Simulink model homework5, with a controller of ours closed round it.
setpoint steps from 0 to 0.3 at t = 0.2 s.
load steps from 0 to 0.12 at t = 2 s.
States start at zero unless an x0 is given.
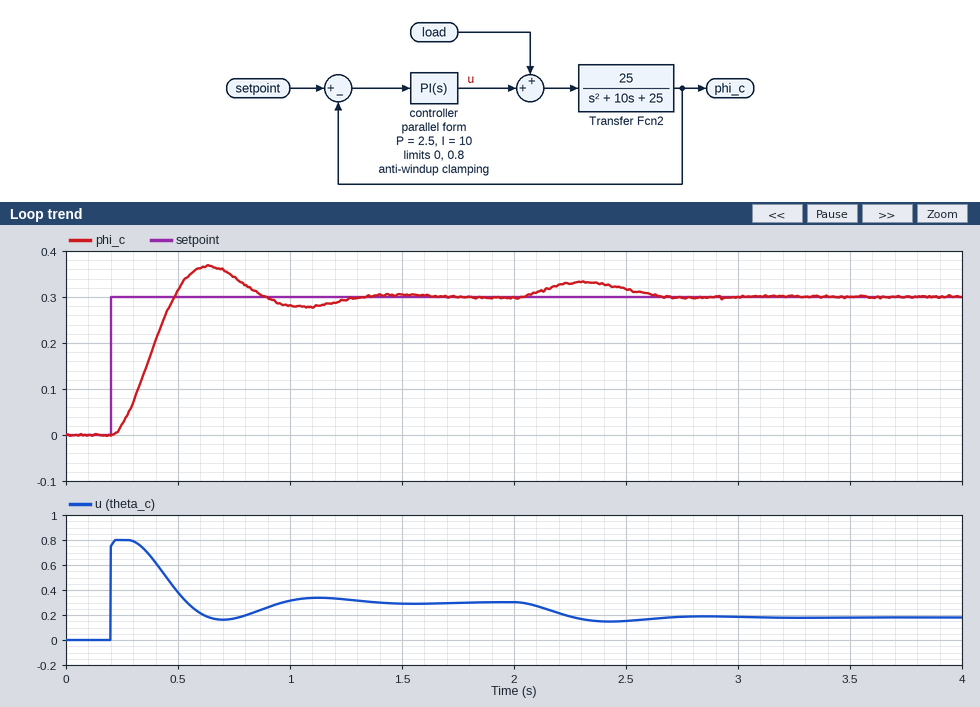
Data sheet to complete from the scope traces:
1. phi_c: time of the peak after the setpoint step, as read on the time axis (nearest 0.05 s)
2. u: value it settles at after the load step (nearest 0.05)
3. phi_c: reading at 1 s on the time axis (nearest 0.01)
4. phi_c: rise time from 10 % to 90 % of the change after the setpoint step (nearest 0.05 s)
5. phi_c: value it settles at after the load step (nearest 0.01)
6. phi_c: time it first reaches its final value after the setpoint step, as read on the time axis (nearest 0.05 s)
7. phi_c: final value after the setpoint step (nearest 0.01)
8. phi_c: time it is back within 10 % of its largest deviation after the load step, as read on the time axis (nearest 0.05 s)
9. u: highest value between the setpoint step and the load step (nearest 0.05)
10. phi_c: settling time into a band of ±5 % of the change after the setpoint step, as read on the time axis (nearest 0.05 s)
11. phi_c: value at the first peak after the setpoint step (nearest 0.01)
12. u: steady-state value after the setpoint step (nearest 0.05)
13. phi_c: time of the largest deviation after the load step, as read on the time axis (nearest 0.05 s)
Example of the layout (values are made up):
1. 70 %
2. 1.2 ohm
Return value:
1. 0.65 s
2. 0.20
3. 0.28
4. 0.20 s
5. 0.30
6. 0.50 s
7. 0.30
8. 2.65 s
9. 0.80
10. 1.15 s
11. 0.37
12. 0.30
13. 2.30 s
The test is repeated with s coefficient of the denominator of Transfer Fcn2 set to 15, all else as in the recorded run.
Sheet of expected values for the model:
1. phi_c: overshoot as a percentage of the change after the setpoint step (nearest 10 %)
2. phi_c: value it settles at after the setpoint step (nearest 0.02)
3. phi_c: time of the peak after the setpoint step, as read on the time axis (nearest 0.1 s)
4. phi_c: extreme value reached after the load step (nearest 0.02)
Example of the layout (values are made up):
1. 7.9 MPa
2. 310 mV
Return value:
1. 20 %
2. 0.30
3. 0.8 s
4. 0.32
